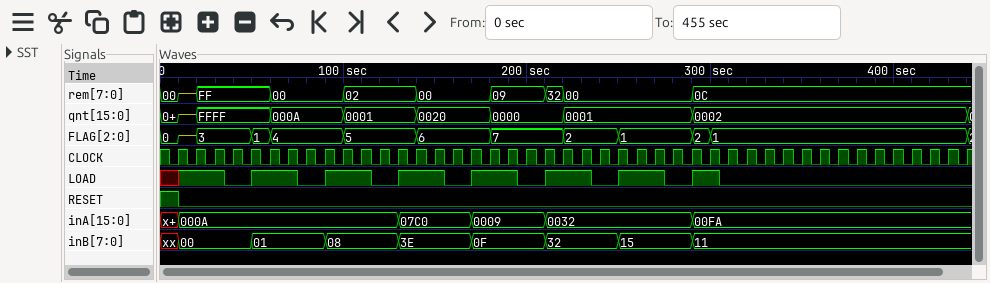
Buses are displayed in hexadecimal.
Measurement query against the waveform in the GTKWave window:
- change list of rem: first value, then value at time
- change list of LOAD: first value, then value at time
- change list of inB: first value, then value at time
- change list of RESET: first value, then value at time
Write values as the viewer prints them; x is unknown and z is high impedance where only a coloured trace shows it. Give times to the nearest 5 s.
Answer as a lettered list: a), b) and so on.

a) 00, z at 10 s, FF at 20 s, 00 at 60 s, 02 at 100 s, 00 at 140 s, 09 at 180 s, 32 at 210 s, 00 at 220 s, 0C at 290 s
b) x, 1 at 10 s, 0 at 35 s, 1 at 50 s, 0 at 75 s, 1 at 90 s, 0 at 115 s, 1 at 130 s, 0 at 155 s, 1 at 170 s, 0 at 195 s, 1 at 210 s, 0 at 235 s, 1 at 250 s, 0 at 275 s, 1 at 290 s, 0 at 305 s
c) xx, 00 at 10 s, 01 at 50 s, 08 at 90 s, 3E at 130 s, 0F at 170 s, 32 at 210 s, 15 at 250 s, 11 at 290 s
d) 1, 0 at 10 s
